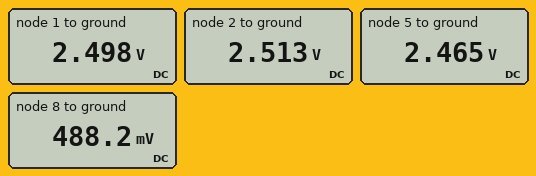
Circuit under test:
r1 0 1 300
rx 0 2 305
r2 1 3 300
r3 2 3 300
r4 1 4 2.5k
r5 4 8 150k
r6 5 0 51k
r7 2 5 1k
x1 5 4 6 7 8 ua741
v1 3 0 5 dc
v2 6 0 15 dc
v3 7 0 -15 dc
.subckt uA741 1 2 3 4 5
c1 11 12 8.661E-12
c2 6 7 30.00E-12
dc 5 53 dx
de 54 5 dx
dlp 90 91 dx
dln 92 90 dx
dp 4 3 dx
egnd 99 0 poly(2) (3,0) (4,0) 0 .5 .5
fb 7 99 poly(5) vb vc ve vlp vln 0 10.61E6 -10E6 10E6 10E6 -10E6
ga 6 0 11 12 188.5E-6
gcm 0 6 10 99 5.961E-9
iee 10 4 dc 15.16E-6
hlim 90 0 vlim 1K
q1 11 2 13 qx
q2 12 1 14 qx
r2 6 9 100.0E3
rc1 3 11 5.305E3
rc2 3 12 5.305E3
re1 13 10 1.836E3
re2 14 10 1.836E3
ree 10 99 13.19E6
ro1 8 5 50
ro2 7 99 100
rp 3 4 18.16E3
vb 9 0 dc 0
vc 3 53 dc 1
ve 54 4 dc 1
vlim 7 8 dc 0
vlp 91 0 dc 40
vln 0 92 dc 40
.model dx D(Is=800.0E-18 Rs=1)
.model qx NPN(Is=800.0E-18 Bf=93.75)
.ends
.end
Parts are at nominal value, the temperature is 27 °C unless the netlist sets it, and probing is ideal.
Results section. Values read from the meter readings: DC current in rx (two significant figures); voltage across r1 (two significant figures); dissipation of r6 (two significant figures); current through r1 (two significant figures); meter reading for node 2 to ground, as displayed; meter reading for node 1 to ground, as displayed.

8.2 mA
2.5 V
120 µW
8.3 mA
2.513 V
2.498 V
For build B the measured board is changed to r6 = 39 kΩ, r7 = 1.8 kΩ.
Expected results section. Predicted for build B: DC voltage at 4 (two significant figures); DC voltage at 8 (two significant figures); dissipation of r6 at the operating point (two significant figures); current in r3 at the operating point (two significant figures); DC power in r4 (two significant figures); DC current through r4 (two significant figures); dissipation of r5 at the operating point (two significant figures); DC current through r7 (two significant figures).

2.4 V
-3.2 V
150 µW
8.3 mA
3.5 µW
38 µA
210 µW
62 µA
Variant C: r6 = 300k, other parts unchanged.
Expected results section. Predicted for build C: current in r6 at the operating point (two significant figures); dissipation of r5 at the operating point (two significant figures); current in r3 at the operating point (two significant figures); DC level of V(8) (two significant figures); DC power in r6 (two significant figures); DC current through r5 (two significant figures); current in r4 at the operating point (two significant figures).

8.4 µA
2.6 µW
8.3 mA
3.1 V
21 µW
4.2 µA
4.1 µA
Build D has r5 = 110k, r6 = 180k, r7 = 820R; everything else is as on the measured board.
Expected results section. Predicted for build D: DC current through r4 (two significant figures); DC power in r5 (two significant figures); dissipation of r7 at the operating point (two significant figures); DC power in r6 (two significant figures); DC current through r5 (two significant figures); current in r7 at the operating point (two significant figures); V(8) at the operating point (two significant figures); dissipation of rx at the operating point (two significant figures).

2.6 µA
810 nW
160 nW
35 µW
2.7 µA
14 µA
2.8 V
21 mW
